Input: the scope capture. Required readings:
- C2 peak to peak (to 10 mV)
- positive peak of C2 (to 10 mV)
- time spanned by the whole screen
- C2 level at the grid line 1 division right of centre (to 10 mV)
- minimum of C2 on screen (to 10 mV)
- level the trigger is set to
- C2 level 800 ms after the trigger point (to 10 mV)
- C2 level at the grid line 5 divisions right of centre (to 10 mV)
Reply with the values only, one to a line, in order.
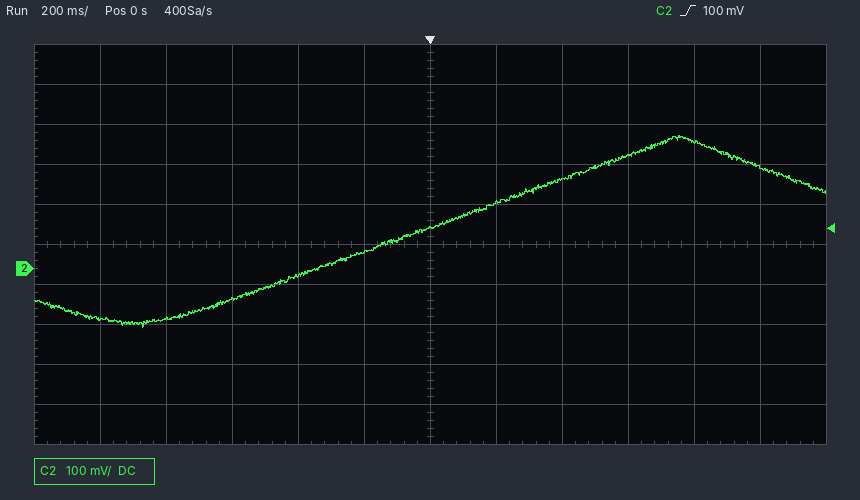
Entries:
480 mV
330 mV
2.4 s
160 mV
-150 mV
100 mV
320 mV
250 mV
